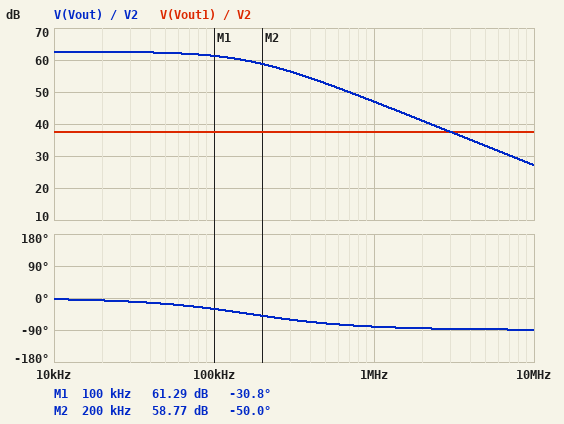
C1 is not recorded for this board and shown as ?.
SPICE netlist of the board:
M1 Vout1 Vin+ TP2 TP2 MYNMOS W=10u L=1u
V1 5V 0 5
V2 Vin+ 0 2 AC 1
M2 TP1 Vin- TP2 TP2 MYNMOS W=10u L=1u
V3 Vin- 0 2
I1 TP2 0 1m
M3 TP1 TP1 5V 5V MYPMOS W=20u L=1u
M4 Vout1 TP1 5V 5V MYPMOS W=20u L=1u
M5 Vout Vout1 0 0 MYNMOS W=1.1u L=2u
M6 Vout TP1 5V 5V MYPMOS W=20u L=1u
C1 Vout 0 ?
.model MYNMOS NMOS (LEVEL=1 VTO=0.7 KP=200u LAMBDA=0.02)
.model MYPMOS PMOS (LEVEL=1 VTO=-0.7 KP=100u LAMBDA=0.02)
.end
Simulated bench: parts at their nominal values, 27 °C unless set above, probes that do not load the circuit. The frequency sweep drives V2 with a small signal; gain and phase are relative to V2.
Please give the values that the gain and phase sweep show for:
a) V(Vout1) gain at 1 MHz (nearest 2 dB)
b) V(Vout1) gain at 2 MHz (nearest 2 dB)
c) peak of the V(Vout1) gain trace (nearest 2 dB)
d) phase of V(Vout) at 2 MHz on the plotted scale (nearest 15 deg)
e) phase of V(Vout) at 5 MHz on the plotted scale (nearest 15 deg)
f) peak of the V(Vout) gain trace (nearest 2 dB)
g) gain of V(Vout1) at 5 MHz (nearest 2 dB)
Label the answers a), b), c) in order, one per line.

a) 38 dB
b) 38 dB
c) 38 dB
d) -90 deg
e) -90 deg
f) 62 dB
g) 38 dB
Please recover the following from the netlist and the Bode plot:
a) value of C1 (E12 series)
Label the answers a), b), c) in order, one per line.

a) 18 pF
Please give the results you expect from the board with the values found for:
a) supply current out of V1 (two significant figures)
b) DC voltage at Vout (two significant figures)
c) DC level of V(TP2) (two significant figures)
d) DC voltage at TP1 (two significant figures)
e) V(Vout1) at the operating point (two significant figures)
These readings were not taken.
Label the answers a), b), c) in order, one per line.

a) 1.5 mA
b) 3.8 V
c) 610 mV
d) 3.6 V
e) 3.6 V
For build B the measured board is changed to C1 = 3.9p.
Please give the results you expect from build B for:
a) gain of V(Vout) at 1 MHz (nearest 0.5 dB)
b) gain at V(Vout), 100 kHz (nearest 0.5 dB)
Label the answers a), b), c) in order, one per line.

a) 58.5 dB
b) 62.5 dB
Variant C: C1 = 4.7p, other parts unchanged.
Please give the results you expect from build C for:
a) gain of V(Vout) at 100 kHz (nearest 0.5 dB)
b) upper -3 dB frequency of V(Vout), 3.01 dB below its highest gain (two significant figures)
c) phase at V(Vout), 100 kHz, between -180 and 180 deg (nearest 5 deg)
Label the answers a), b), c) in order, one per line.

a) 62.5 dB
b) 640 kHz
c) -10 deg
